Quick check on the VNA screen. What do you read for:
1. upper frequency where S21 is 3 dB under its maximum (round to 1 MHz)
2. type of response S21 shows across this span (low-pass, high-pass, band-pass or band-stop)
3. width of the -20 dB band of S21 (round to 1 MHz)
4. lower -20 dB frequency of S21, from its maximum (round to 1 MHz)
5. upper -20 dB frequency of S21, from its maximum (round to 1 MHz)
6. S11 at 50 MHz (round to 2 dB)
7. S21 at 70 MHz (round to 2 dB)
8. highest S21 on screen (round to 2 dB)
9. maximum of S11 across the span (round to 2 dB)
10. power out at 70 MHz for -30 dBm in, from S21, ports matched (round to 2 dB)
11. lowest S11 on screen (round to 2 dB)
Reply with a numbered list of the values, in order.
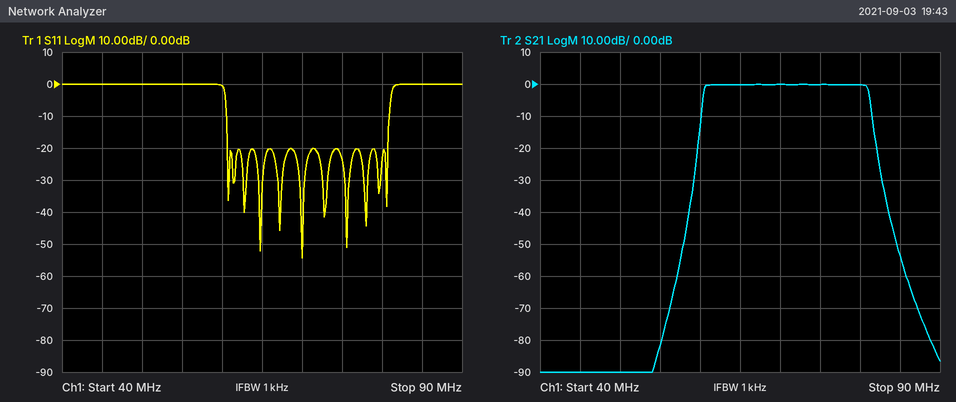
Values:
1. 81 MHz
2. band-pass
3. 22 MHz
4. 60 MHz
5. 82 MHz
6. 0 dB
7. 0 dB
8. 0 dB
9. 0 dB
10. -30 dBm
11. -54 dB
